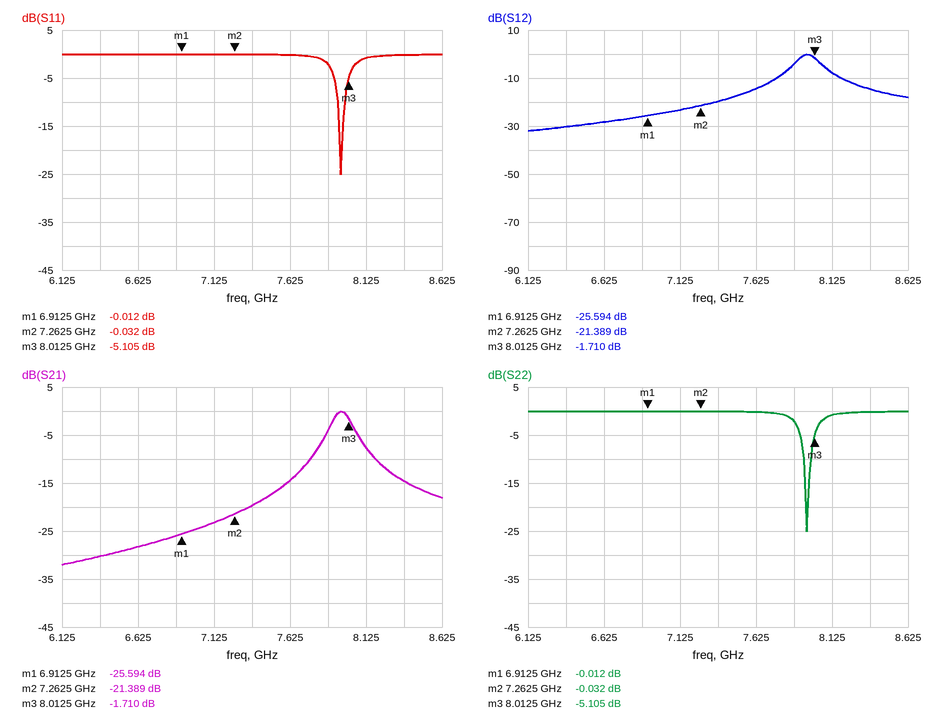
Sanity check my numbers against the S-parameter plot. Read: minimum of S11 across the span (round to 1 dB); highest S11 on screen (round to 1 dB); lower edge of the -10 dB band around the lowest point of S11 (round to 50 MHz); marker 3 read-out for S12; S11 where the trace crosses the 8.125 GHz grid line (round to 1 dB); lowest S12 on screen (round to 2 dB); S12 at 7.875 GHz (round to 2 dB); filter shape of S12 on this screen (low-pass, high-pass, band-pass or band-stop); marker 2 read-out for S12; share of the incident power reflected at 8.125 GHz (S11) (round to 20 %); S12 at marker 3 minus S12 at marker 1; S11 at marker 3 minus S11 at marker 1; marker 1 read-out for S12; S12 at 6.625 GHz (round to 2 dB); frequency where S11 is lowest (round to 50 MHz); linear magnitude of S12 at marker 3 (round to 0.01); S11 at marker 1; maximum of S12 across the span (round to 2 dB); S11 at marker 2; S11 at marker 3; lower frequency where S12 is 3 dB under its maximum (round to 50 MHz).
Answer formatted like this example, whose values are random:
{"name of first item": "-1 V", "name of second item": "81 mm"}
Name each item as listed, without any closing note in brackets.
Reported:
{"minimum of S11 across the span": "-25 dB", "highest S11 on screen": "0 dB", "lower edge of the -10 dB band around the lowest point of S11": "7.95 GHz", "marker 3 read-out for S12": "-1.710 dB", "S11 where the trace crosses the 8.125 GHz grid line": "-1 dB", "lowest S12 on screen": "-32 dB", "S12 at 7.875 GHz": "-4 dB", "filter shape of S12 on this screen": "band-pass", "marker 2 read-out for S12": "-21.389 dB", "share of the incident power reflected at 8.125 GHz (S11)": "80 %", "S12 at marker 3 minus S12 at marker 1": "23.884 dB", "S11 at marker 3 minus S11 at marker 1": "-5.093 dB", "marker 1 read-out for S12": "-25.594 dB", "S12 at 6.625 GHz": "-28 dB", "frequency where S11 is lowest": "7.95 GHz", "linear magnitude of S12 at marker 3": "0.82", "S11 at marker 1": "-0.012 dB", "maximum of S12 across the span": "0 dB", "S11 at marker 2": "-0.032 dB", "S11 at marker 3": "-5.105 dB", "lower frequency where S12 is 3 dB under its maximum": "7.90 GHz"}
